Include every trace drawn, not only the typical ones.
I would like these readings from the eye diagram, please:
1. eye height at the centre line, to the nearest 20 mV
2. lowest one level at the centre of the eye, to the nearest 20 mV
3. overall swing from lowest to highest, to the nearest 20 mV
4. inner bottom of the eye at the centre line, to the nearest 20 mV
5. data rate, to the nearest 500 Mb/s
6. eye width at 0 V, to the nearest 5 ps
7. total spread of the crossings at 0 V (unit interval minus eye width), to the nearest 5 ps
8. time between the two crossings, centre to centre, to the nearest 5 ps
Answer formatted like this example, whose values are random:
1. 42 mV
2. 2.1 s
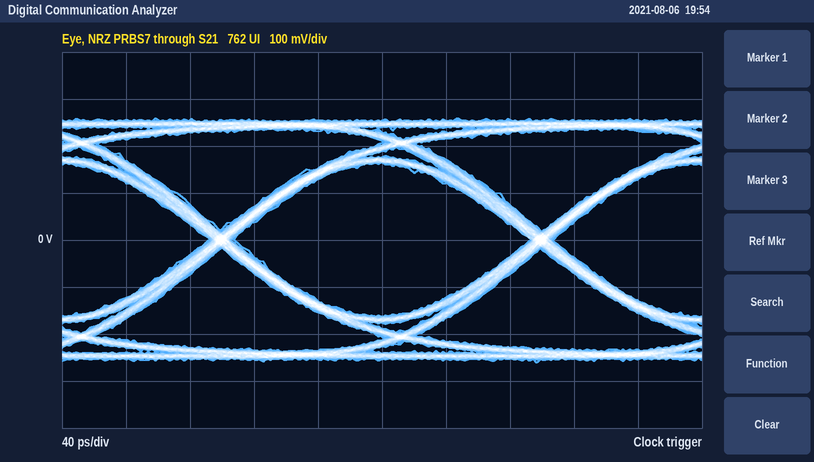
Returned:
1. 320 mV
2. 160 mV
3. 520 mV
4. -160 mV
5. 5.0 Gb/s
6. 185 ps
7. 15 ps
8. 200 ps
